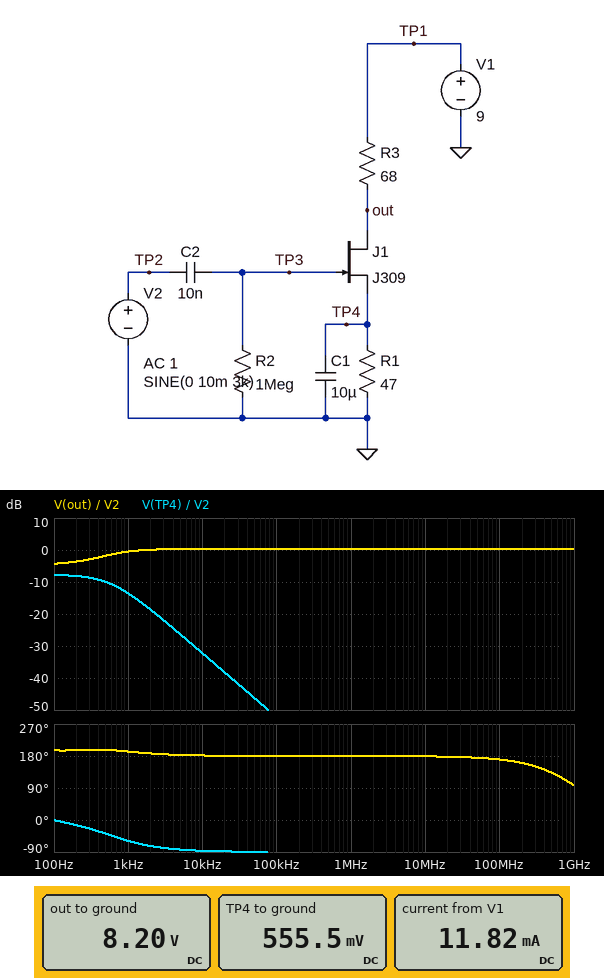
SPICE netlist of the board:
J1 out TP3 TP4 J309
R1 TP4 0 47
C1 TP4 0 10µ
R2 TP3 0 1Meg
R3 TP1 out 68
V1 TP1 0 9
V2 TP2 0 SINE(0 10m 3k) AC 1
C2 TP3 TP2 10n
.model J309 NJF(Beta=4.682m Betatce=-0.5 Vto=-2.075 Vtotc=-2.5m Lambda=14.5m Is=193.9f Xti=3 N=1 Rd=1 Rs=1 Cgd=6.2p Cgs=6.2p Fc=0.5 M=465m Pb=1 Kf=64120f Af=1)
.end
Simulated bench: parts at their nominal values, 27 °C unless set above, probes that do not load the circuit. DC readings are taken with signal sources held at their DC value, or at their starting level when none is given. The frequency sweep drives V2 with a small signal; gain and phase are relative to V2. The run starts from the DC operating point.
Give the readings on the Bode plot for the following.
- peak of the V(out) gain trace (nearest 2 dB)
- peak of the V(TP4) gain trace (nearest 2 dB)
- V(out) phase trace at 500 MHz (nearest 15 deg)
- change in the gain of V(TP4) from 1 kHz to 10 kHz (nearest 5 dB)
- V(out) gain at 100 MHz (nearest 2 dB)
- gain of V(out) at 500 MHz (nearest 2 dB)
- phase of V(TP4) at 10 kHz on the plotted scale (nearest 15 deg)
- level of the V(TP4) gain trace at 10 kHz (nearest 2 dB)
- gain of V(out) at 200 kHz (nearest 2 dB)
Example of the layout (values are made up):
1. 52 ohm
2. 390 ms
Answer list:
1. 0 dB
2. -8 dB
3. 135 deg
4. -20 dB
5. 0 dB
6. 0 dB
7. -90 deg
8. -32 dB
9. 0 dB
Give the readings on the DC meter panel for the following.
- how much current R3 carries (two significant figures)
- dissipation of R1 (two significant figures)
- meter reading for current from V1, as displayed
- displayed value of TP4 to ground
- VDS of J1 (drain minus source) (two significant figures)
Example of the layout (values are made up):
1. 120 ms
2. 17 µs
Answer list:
1. 12 mA
2. 6.6 mW
3. 11.82 mA
4. 555.5 mV
5. 7.6 V
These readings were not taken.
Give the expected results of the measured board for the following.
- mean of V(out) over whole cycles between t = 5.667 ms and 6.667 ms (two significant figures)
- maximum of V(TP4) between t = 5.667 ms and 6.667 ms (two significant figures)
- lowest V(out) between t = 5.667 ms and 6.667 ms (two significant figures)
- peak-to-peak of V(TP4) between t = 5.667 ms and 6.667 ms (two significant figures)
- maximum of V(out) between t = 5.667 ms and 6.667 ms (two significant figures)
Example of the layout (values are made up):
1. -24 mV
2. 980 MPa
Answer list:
1. 8.2 V
2. 560 mV
3. 8.2 V
4. 1.6 mV
5. 8.2 V
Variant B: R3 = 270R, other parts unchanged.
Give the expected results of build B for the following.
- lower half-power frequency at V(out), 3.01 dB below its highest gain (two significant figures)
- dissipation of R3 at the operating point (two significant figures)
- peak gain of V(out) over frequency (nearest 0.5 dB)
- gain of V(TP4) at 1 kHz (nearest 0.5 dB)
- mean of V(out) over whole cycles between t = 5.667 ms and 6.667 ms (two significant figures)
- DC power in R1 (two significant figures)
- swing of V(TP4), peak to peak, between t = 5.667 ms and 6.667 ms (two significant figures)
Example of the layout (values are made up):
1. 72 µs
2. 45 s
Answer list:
1. 310 Hz
2. 36 mW
3. 12.0 dB
4. -14.0 dB
5. 5.9 V
6. 6.3 mW
7. 1.5 mV
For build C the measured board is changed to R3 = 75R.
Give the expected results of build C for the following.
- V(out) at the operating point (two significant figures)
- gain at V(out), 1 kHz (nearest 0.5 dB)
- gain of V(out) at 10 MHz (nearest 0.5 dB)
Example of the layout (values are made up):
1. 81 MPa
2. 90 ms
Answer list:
1. 8.1 V
2. 0.5 dB
3. 1.0 dB
